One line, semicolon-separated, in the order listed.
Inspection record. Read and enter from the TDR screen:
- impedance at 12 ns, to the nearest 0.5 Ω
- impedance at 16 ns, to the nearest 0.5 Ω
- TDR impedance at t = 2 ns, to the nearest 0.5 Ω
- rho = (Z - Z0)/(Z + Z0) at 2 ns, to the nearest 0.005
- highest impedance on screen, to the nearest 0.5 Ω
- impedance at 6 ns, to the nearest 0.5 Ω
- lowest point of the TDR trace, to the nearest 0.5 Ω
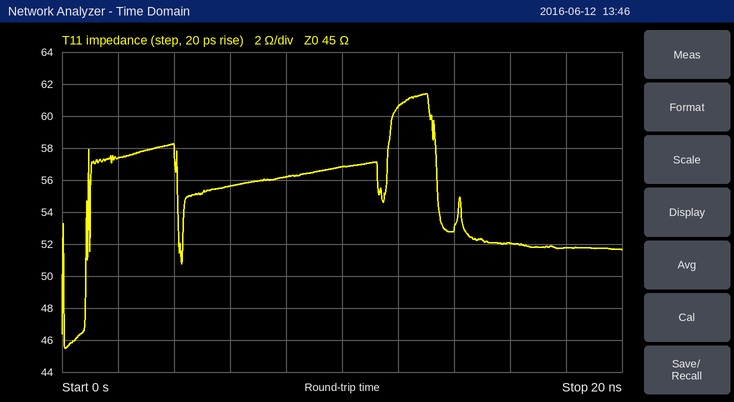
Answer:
60.5 Ω; 52.0 Ω; 57.5 Ω; +0.120; 61.5 Ω; 55.5 Ω; 45.5 Ω
